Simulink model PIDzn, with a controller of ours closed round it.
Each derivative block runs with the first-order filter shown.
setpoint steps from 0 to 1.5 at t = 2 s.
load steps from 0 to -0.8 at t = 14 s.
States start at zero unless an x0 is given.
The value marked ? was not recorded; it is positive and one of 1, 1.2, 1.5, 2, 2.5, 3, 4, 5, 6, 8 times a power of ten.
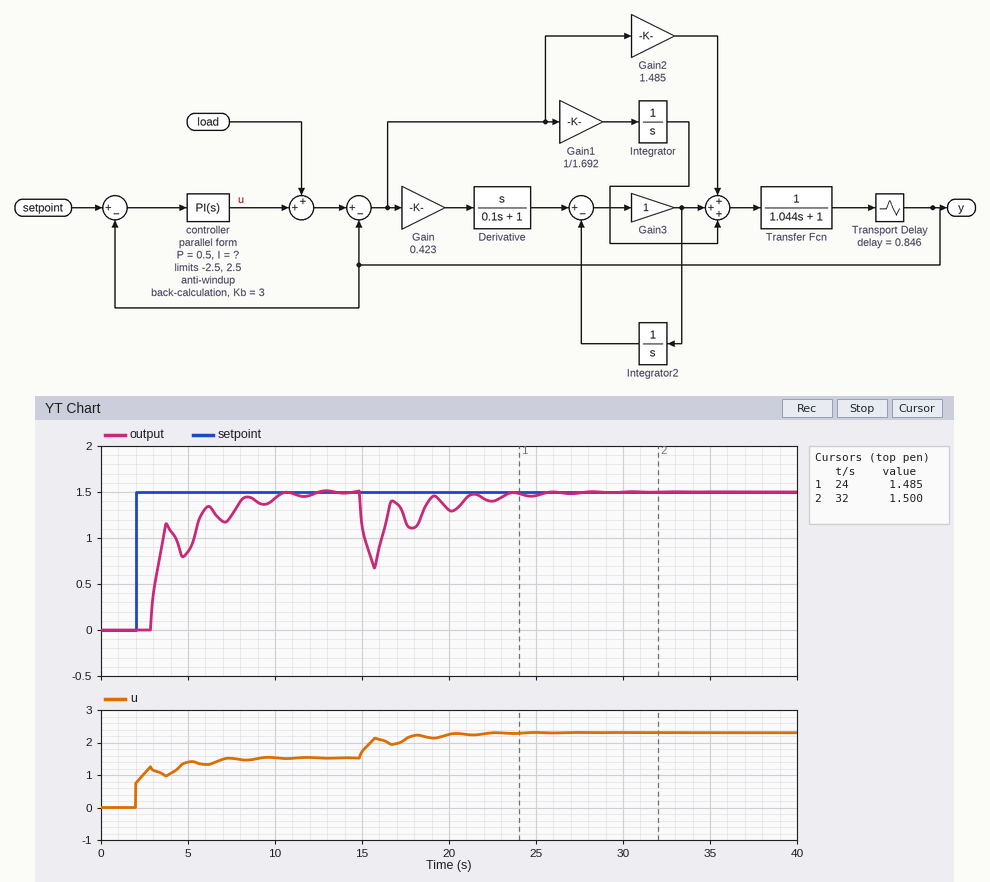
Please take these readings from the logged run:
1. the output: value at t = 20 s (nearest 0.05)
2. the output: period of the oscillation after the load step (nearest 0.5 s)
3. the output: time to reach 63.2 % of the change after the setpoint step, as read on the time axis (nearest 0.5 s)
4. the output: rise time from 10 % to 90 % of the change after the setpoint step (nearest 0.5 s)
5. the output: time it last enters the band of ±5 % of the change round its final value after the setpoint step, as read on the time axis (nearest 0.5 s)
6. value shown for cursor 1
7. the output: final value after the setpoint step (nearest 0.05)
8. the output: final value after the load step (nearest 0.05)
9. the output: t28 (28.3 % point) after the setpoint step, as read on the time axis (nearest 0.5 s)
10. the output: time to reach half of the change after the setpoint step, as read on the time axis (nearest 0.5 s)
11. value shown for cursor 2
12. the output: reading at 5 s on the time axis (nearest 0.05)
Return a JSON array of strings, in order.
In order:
["1.30", "2.0 s", "3.5 s", "5.0 s", "10.0 s", "1.485", "1.50", "1.50", "3.0 s", "3.5 s", "1.500", "0.85"]
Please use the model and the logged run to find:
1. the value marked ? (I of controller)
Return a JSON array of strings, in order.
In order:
["0.4"]
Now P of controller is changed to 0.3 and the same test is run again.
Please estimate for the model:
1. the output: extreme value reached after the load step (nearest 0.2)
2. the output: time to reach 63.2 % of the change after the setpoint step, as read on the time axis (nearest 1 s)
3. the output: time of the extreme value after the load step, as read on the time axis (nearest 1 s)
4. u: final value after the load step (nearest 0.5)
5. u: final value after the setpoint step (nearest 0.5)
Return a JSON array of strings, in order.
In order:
["0.6", "5 s", "16 s", "2.5", "1.5"]
